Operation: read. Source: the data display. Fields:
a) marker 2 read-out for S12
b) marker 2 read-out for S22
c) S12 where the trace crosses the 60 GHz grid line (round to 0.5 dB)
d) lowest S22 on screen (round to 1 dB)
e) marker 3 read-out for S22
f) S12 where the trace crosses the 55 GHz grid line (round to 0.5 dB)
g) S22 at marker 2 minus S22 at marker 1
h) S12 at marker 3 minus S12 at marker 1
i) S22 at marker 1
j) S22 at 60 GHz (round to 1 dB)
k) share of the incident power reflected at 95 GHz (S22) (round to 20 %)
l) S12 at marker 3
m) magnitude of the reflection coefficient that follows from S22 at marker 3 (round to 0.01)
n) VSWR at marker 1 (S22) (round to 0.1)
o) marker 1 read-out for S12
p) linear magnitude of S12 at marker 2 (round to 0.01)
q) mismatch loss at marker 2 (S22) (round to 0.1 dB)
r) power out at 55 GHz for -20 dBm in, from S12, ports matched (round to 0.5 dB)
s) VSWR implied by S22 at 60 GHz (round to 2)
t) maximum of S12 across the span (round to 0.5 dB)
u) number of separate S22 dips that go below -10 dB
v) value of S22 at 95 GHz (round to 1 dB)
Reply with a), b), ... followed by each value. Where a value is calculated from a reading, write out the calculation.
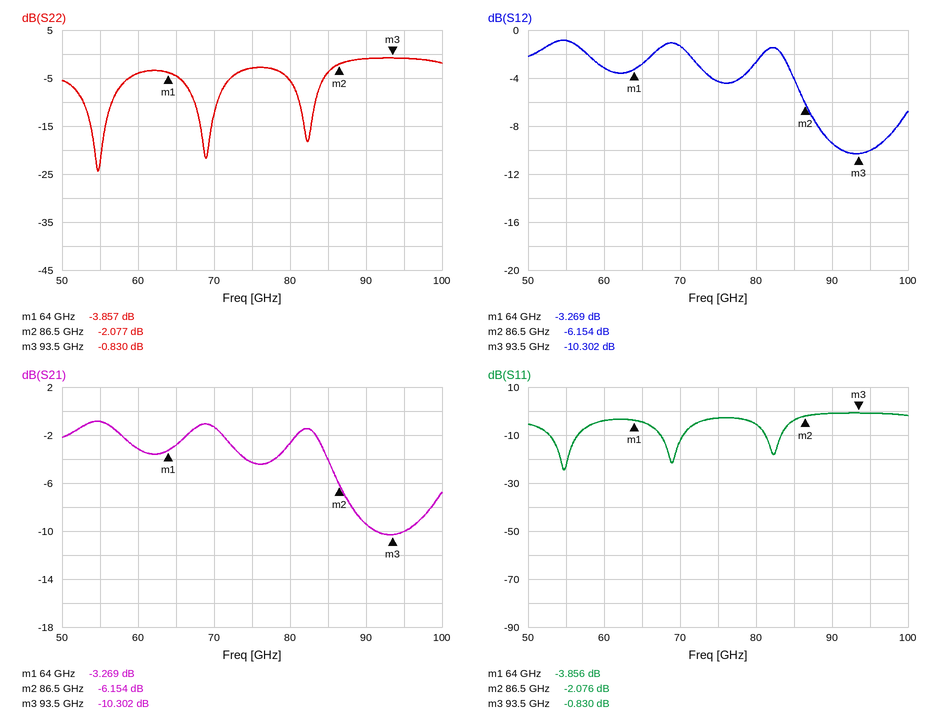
a) -6.154 dB
b) -2.077 dB
c) -3.0 dB
d) -24 dB
e) -0.830 dB
f) -1.0 dB
g) -2.077 − (-3.857) = 1.780 dB
h) -10.302 − (-3.269) = -7.033 dB
i) -3.857 dB
j) -4 dB
k) 10^(-1/10) ≈ 79.4 %, so 80 % to the nearest 20 %
l) -10.302 dB
m) 10^(-0.83/20) ≈ 0.91
n) (1 + 0.6414)/(1 − 0.6414) ≈ 4.6
o) -3.269 dB
p) 10^(-6.154/20) ≈ 0.49
q) −10 log10(1 − 10^(-2.077/10)) ≈ 4.2 dB
r) -20 dBm + (-1.0 dB) = -21.0 dBm
s) |Γ| = 10^(-4/20) = 0.6310; VSWR = (1 + 0.6310)/(1 − 0.6310) ≈ 4
t) -1.0 dB
u) 3
v) -1 dB
